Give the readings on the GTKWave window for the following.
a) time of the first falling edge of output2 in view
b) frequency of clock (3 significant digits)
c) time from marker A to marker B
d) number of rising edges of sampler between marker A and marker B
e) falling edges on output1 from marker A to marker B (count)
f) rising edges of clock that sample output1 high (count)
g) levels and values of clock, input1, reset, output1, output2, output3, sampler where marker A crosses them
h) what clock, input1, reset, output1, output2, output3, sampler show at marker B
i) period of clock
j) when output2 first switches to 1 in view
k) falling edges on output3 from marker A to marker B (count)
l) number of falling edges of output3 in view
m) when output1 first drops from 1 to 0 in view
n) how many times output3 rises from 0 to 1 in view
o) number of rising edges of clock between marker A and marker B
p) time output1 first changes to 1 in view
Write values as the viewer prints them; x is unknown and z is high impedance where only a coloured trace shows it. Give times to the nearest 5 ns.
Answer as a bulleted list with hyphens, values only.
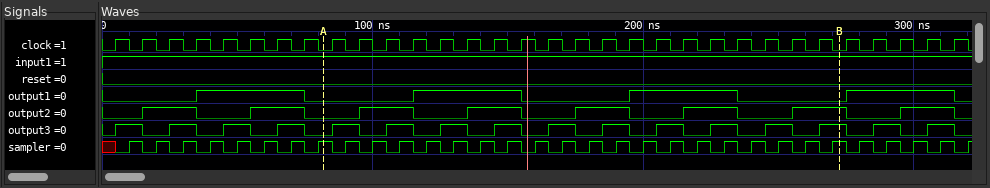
- 35 ns
- 100 MHz
- 190 ns
- 19
- 2
- 16
- clock=0, input1=1, reset=0, output1=0, output2=0, output3=0, sampler=1
- clock=0, input1=1, reset=0, output1=0, output2=1, output3=1, sampler=1
- 10 ns
- 15 ns
- 9
- 16
- 75 ns
- 16
- 19
- 35 ns
